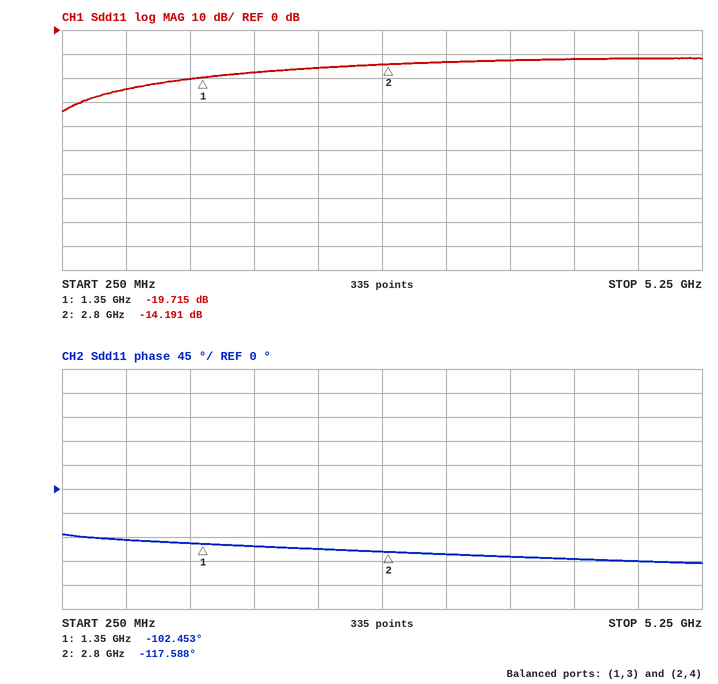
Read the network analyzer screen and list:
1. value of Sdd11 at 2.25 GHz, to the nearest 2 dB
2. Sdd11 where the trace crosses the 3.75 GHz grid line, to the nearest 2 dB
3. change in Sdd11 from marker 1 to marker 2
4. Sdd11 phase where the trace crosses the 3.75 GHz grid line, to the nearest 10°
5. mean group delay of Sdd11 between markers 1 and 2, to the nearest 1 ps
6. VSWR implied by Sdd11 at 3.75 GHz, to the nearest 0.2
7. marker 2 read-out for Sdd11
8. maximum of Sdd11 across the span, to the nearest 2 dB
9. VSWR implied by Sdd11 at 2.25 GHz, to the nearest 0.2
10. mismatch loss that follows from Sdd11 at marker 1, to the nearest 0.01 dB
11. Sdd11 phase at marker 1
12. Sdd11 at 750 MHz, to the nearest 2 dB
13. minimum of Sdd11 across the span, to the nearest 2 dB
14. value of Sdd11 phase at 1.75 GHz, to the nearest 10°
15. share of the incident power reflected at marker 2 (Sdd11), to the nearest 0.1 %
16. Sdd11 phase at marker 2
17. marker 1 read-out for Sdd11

-16 dB
-12 dB
5.524 dB
-130°
29 ps
1.6
-14.191 dB
-12 dB
1.4
0.05 dB
-102.453°
-24 dB
-34 dB
-110°
3.8 %
-117.588°
-19.715 dB
